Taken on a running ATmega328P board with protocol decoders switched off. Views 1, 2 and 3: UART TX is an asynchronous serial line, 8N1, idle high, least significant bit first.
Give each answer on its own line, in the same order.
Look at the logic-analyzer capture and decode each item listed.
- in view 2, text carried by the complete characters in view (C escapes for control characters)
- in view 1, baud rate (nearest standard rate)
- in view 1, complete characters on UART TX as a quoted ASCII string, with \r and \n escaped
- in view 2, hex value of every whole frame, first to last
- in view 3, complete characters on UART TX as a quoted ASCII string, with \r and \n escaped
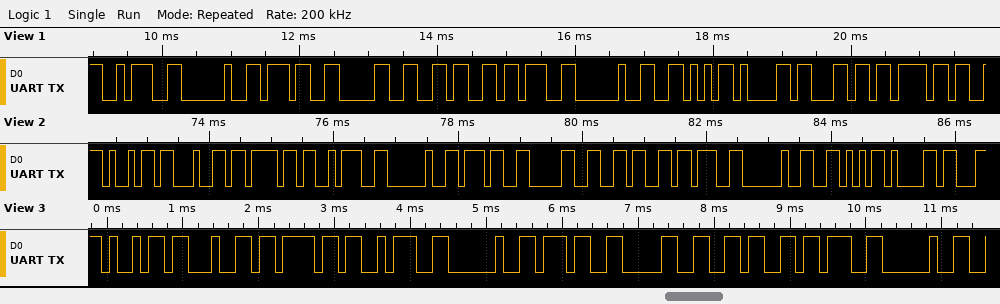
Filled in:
"ido: 706; Va"
9600 baud
": 706; Valo"
69 64 6F 3A 20 37 30 36 3B 20 56 61
"ido: 706; "
